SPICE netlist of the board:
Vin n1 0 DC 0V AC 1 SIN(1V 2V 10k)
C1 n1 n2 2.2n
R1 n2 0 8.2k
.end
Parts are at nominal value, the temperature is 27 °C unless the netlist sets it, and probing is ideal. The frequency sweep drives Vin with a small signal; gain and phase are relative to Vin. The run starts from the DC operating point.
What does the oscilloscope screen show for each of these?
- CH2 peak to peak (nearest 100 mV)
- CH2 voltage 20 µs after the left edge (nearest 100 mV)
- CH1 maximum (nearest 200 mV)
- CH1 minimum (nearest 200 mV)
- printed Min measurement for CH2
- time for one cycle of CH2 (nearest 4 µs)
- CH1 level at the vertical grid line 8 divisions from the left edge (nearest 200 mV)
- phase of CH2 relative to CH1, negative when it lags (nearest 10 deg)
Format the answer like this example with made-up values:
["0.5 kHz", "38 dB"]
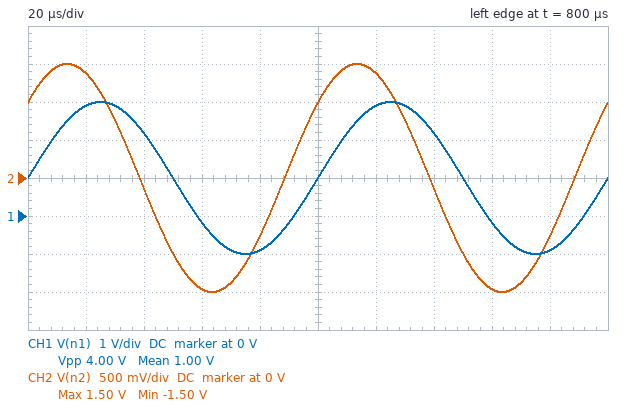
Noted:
["3.0 V", "1.4 V", "3.0 V", "-1.0 V", "-1.50 V", "100 µs", "-200 mV", "40 deg"]
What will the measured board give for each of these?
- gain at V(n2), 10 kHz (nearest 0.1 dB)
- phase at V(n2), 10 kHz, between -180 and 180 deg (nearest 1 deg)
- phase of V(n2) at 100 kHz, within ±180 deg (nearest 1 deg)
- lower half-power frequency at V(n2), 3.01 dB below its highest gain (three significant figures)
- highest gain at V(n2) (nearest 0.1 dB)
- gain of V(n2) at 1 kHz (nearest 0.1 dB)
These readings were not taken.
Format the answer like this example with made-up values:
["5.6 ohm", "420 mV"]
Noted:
["-2.5 dB", "41 deg", "5 deg", "8.82 kHz", "0 dB", "-19.0 dB"]
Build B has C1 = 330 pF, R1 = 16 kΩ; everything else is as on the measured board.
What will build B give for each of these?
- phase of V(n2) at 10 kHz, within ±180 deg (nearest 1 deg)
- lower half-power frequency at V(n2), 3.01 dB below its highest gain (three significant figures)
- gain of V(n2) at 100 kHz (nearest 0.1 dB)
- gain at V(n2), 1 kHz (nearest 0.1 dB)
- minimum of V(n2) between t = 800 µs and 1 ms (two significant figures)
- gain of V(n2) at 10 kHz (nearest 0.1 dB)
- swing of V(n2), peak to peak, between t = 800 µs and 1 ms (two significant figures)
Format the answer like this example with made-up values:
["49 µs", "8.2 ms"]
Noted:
["72 deg", "30.1 kHz", "-0.4 dB", "-29.6 dB", "-630 mV", "-10.0 dB", "1.3 V"]
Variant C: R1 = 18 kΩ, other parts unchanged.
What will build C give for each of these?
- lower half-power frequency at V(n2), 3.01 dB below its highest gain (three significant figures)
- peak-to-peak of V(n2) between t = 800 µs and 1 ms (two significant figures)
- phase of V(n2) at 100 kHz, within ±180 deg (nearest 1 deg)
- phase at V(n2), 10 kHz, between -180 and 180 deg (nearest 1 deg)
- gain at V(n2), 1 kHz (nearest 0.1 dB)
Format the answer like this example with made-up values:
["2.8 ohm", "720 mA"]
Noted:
["4.02 kHz", "3.7 V", "2 deg", "22 deg", "-12.3 dB"]
